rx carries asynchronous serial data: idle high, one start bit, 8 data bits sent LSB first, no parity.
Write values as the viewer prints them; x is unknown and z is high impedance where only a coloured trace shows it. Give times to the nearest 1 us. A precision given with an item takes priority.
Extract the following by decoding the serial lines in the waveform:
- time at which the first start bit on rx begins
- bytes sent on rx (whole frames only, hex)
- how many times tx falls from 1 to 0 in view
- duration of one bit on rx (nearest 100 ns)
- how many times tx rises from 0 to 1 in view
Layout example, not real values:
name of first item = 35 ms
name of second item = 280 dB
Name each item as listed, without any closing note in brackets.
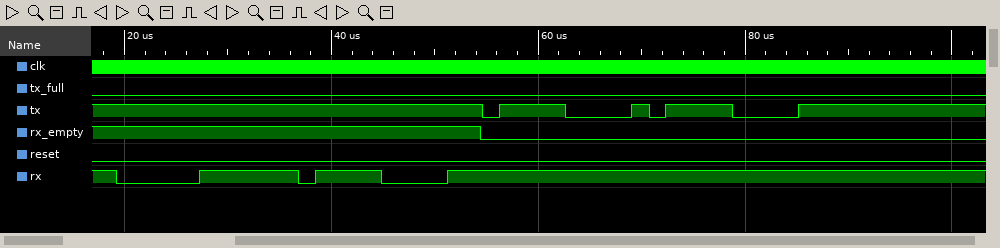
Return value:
time at which the first start bit on rx begins = 19 us
bytes sent on rx = F0, 0F
how many times tx falls from 1 to 0 in view = 4
duration of one bit on rx = 1600 ns
how many times tx rises from 0 to 1 in view = 4
